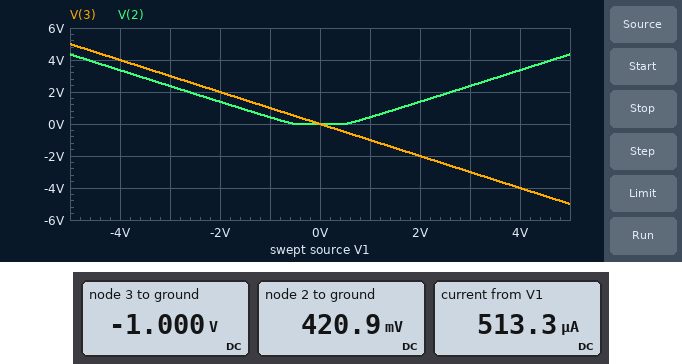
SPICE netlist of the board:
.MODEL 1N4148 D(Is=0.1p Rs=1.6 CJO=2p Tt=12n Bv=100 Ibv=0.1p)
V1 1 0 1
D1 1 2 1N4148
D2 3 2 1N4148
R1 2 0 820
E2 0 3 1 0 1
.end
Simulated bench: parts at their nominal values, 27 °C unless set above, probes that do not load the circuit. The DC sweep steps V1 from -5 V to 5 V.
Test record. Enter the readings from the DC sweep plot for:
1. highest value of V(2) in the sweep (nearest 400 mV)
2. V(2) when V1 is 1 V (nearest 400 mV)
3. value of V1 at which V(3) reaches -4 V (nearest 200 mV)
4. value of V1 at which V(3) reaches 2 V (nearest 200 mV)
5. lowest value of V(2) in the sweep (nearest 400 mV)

4.4 V
400 mV
4.0 V
-2.0 V
0 V
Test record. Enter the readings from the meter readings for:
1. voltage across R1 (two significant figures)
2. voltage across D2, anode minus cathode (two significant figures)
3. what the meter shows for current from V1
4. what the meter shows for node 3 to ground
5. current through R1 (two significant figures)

420 mV
-1.4 V
513.3 µA
-1.000 V
510 µA
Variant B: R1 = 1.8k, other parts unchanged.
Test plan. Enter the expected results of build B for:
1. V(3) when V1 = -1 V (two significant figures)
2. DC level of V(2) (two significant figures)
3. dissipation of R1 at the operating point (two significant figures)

1.0 V
440 mV
110 µW
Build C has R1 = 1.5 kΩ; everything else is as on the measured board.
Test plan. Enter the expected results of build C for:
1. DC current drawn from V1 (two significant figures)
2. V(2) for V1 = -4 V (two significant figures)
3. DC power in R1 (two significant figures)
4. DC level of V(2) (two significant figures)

290 µA
3.4 V
130 µW
440 mV
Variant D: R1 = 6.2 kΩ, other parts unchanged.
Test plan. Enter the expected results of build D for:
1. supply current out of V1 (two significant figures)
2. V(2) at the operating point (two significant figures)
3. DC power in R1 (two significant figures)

76 µA
470 mV
36 µW
